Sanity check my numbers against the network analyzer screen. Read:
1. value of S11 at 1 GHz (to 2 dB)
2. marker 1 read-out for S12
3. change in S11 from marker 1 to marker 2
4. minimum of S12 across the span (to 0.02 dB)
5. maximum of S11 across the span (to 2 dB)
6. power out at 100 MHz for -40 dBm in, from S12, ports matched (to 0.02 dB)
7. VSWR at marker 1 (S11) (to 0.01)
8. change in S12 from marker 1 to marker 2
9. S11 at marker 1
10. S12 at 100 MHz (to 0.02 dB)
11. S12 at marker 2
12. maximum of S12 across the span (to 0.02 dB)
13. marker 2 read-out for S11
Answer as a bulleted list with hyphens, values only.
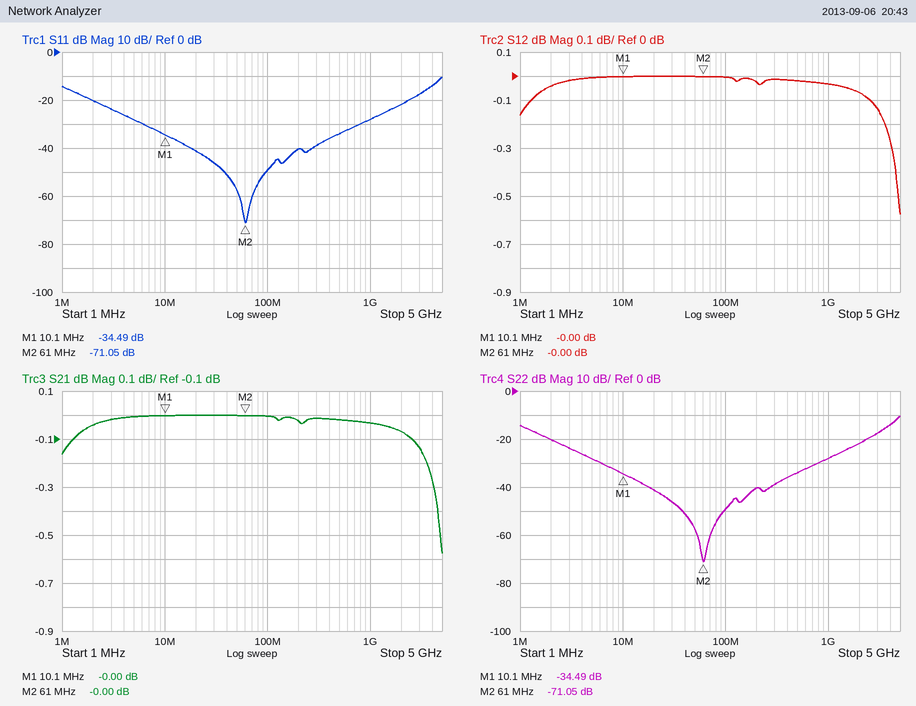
- -28 dB
- -0.00 dB
- -36.56 dB
- -0.58 dB
- -10 dB
- -40.00 dBm
- 1.04
- 0.00 dB
- -34.49 dB
- 0.00 dB
- -0.00 dB
- 0.00 dB
- -71.05 dB
